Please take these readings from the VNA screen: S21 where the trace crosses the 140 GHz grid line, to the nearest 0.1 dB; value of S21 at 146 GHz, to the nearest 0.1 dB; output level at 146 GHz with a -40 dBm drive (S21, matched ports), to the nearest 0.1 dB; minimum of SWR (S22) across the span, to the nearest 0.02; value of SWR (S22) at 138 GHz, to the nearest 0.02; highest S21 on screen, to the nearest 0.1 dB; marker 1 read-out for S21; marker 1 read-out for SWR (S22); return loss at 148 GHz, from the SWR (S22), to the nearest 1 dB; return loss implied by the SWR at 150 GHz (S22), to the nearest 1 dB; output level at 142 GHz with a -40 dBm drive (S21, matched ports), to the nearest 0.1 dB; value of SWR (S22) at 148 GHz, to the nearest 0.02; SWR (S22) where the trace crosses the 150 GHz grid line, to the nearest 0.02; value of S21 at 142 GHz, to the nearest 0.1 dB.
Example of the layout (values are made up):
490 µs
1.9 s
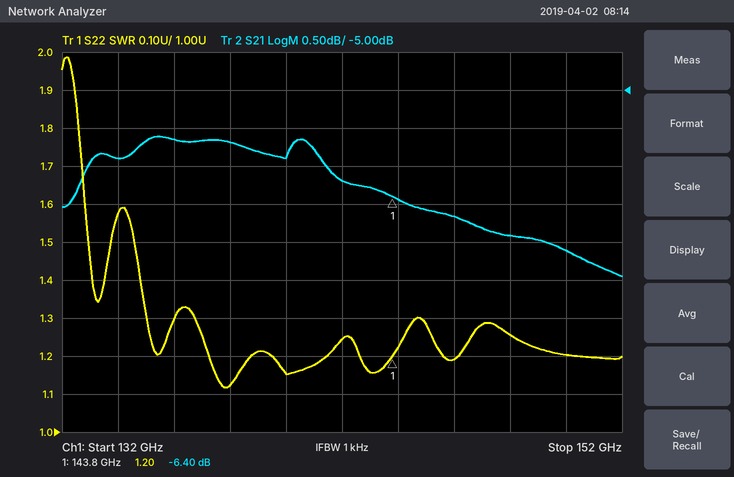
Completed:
-5.9 dB
-6.7 dB
-46.7 dBm
1.12
1.12
-5.6 dB
-6.40 dB
1.20
19 dB
21 dB
-46.2 dBm
1.26
1.20
-6.2 dB
